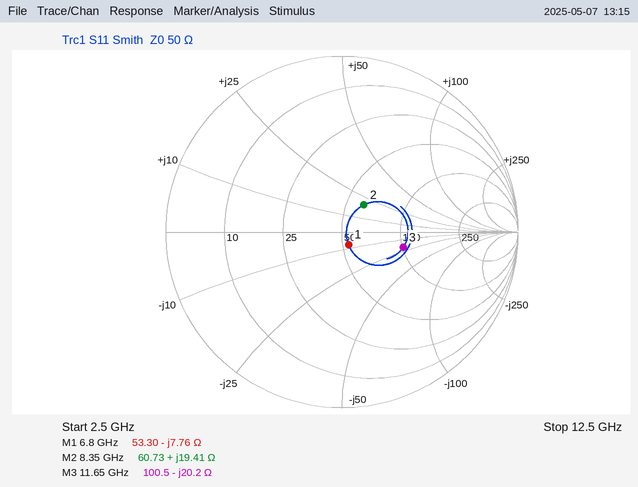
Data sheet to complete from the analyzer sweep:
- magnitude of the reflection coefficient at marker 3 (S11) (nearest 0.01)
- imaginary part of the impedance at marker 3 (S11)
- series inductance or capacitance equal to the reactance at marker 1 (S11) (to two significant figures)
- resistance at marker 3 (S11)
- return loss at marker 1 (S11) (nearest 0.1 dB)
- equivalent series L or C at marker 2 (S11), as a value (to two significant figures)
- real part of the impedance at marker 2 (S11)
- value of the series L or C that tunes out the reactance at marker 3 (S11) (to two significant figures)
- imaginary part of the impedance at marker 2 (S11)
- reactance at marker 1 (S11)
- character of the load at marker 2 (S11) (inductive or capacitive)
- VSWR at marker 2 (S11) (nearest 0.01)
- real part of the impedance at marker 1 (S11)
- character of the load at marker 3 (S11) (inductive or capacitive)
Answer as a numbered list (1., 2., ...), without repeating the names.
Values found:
1. 0.36
2. -20.2 Ω
3. 3.0 pF
4. 100.5 Ω
5. 21.8 dB
6. 370 pH
7. 60.73 Ω
8. 280 pH
9. +19.41 Ω
10. -7.76 Ω
11. inductive
12. 1.49
13. 53.30 Ω
14. capacitive
